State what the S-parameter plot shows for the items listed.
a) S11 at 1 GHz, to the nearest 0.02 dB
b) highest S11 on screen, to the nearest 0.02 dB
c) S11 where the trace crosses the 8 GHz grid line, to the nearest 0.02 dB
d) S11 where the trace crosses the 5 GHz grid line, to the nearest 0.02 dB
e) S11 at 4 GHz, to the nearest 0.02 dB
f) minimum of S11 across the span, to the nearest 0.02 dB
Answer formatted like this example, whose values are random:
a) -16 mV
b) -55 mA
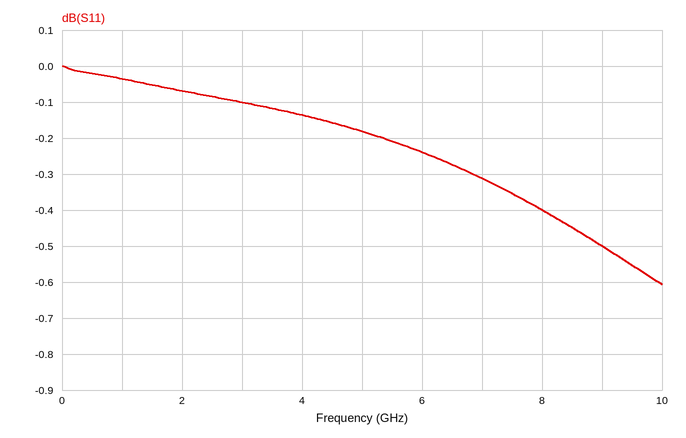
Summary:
a) -0.04 dB
b) 0.00 dB
c) -0.40 dB
d) -0.18 dB
e) -0.14 dB
f) -0.60 dB
